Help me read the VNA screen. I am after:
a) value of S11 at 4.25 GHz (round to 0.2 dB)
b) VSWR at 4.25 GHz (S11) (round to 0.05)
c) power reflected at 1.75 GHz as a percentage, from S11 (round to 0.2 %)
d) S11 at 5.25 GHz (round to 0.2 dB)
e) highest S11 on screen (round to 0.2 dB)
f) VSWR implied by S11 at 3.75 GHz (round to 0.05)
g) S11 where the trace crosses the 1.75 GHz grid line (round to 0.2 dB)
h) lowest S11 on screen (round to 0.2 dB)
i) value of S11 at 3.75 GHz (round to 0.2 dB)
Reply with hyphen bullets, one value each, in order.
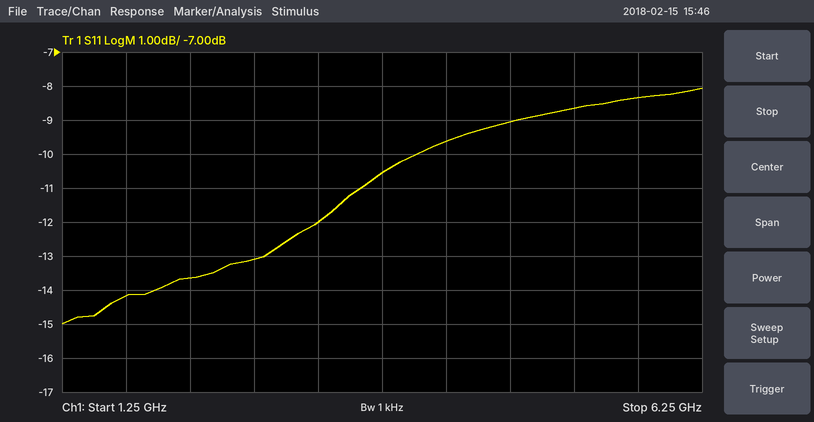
- -9.6 dB
- 2.00
- 3.8 %
- -8.6 dB
- -8.0 dB
- 1.85
- -14.2 dB
- -15.0 dB
- -10.6 dB
